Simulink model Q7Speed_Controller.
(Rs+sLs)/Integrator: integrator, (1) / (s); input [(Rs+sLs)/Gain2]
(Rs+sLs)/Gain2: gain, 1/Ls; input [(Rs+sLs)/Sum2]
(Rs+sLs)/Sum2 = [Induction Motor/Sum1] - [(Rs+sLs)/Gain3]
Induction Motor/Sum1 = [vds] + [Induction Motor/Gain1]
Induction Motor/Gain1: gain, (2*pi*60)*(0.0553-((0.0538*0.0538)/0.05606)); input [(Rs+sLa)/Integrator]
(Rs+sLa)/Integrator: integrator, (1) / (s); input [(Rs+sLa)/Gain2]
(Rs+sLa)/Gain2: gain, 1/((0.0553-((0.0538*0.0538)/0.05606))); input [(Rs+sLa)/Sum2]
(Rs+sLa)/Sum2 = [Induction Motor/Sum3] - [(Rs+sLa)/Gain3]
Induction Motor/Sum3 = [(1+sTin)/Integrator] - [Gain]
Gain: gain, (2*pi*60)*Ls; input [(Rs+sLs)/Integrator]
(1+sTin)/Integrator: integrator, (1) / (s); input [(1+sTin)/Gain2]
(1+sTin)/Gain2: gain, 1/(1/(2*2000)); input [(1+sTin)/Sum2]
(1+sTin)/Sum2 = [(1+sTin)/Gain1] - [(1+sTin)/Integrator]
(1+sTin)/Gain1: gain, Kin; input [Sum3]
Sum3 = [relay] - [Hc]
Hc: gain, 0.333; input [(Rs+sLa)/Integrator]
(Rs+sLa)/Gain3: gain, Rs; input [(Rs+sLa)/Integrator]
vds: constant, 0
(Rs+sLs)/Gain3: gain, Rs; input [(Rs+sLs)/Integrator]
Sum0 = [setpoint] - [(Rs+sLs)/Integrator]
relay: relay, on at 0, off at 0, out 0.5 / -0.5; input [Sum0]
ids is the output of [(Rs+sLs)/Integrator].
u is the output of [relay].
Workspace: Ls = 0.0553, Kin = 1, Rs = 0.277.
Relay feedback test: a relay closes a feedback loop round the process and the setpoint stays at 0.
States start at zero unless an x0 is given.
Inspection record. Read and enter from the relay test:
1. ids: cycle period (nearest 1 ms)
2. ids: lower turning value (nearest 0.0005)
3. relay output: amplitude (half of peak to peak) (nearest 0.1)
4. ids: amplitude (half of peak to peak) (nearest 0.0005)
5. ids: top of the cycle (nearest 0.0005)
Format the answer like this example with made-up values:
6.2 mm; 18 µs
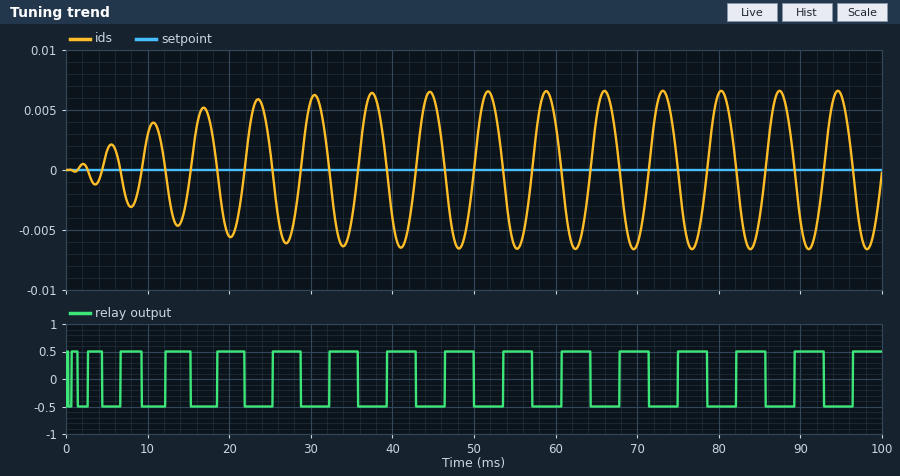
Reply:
7 ms; -0.0065; 0.5; 0.0065; 0.0065
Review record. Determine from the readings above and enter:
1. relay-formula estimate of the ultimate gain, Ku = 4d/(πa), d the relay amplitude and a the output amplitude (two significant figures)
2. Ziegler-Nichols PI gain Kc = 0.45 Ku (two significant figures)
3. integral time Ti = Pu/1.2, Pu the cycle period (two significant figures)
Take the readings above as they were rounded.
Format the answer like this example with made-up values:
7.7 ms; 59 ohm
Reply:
98; 44; 5.8 ms
